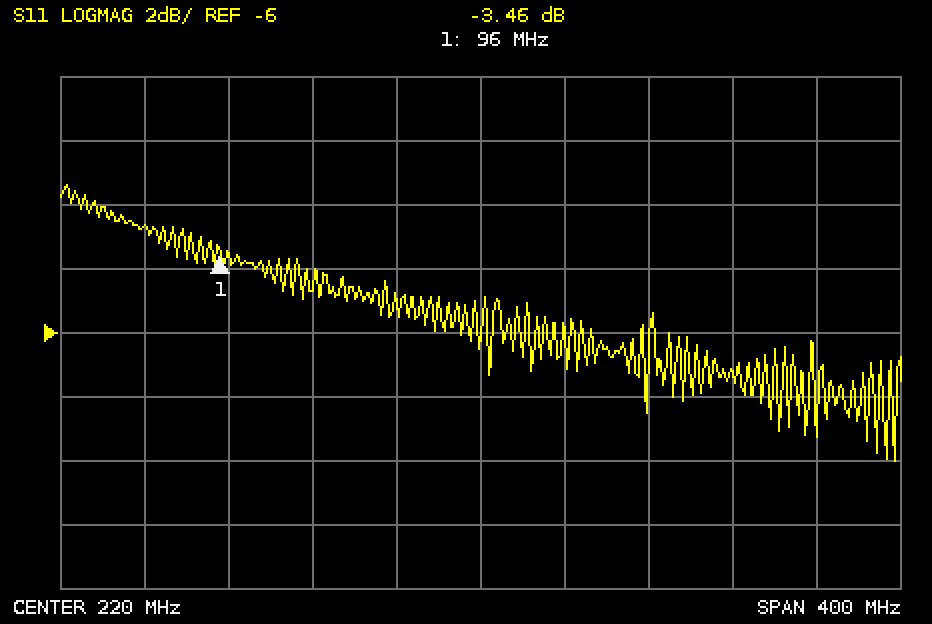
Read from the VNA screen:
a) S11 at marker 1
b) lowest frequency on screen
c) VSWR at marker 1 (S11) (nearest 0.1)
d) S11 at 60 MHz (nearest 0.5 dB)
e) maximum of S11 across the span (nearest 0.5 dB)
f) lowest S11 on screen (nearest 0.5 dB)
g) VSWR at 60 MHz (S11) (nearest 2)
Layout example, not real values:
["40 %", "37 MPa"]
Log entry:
["-3.46 dB", "20 MHz", "5.1", "-2.5 dB", "-1.5 dB", "-10.0 dB", "6"]
